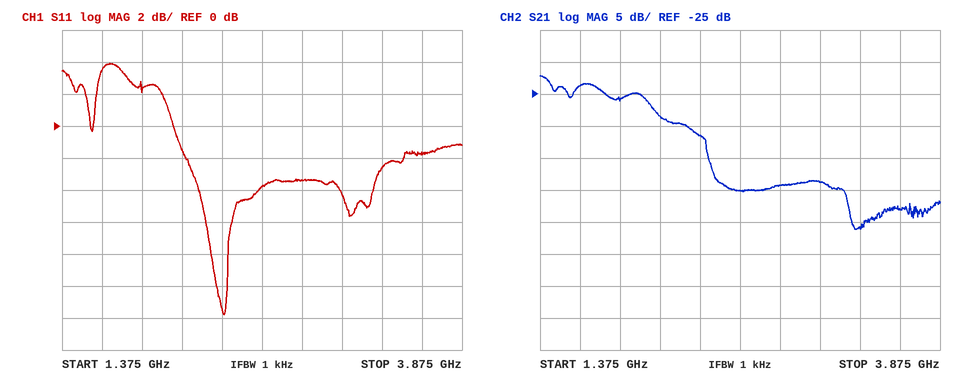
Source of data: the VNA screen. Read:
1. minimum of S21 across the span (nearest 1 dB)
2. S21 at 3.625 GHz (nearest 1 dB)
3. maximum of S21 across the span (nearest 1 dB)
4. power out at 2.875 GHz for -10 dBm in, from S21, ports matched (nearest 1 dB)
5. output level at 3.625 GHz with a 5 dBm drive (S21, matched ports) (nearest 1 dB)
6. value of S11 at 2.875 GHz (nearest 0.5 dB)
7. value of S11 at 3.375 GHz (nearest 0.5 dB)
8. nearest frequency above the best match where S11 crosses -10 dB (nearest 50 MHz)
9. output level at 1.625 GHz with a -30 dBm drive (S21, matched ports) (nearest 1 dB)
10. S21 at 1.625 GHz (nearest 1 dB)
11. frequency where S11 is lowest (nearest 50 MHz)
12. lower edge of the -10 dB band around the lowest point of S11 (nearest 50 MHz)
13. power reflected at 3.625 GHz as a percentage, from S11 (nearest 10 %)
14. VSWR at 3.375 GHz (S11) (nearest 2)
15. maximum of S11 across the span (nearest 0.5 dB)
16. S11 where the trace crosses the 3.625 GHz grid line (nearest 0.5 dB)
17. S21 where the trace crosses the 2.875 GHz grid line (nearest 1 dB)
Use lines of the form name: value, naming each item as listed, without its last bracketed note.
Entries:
minimum of S21 across the span: -46 dB
S21 at 3.625 GHz: -43 dB
maximum of S21 across the span: -22 dB
power out at 2.875 GHz for -10 dBm in, from S21, ports matched: -49 dBm
output level at 3.625 GHz with a 5 dBm drive (S21, matched ports): -38 dBm
value of S11 at 2.875 GHz: -3.5 dB
value of S11 at 3.375 GHz: -2.5 dB
nearest frequency above the best match where S11 crosses -10 dB: 2.40 GHz
output level at 1.625 GHz with a -30 dBm drive (S21, matched ports): -54 dBm
S21 at 1.625 GHz: -24 dB
frequency where S11 is lowest: 2.40 GHz
lower edge of the -10 dB band around the lowest point of S11: 2.35 GHz
power reflected at 3.625 GHz as a percentage, from S11: 70 %
VSWR at 3.375 GHz (S11): 6
maximum of S11 across the span: 4.0 dB
S11 where the trace crosses the 3.625 GHz grid line: -1.5 dB
S21 where the trace crosses the 2.875 GHz grid line: -39 dB
